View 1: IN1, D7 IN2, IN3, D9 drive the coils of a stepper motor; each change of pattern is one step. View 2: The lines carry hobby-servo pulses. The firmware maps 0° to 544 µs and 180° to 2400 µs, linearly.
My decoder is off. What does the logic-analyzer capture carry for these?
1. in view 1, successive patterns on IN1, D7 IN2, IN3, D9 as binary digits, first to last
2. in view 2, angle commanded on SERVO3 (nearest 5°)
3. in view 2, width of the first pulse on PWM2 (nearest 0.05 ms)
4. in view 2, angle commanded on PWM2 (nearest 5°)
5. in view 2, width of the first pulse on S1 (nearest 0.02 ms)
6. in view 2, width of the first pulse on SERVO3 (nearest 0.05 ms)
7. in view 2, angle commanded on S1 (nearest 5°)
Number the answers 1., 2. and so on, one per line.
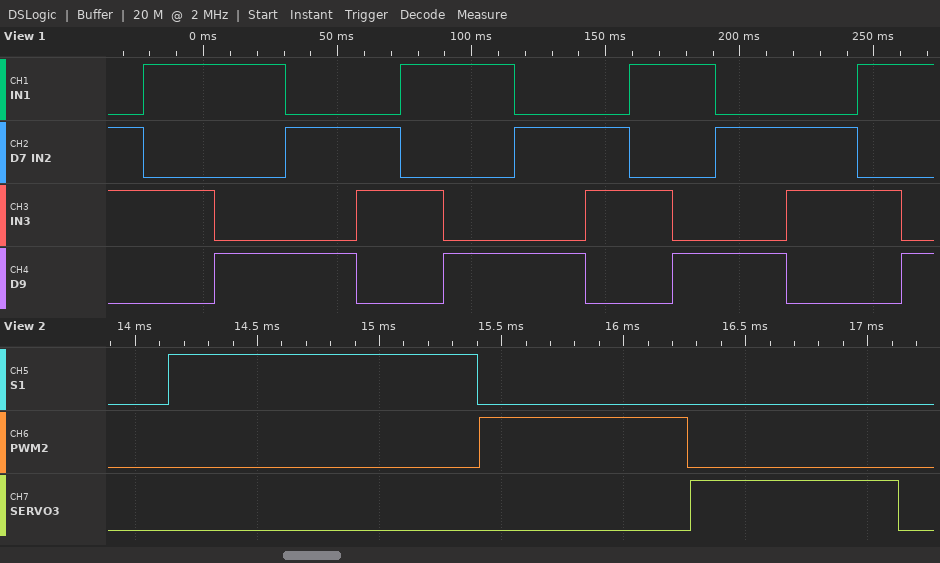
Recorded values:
1. 0110 1010 1001 0101 0110 1010 1001 0101 0110 1010 1001 0101 0110 1010 1001
2. 30°
3. 0.85 ms
4. 30°
5. 1.26 ms
6. 0.85 ms
7. 70°
